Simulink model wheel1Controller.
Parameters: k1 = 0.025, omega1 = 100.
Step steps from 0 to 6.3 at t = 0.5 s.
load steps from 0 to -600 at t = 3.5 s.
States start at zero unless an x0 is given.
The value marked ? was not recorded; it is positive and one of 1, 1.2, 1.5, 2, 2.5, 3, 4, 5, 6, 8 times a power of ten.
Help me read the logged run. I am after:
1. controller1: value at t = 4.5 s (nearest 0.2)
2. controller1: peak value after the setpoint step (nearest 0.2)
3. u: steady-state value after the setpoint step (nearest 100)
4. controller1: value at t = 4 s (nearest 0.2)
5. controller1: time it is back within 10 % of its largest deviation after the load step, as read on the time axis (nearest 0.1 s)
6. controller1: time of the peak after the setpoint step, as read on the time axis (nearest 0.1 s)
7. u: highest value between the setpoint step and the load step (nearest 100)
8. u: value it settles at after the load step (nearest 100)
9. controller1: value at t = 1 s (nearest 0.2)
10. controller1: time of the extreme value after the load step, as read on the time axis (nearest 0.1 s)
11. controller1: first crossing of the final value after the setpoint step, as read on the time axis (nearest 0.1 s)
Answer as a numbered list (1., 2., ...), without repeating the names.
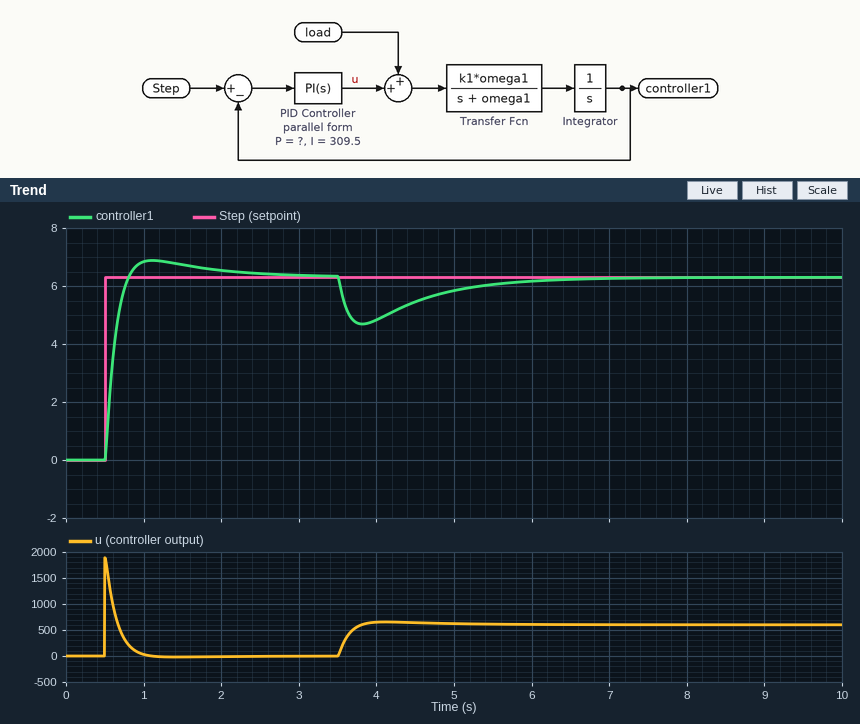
1. 5.4
2. 6.8
3. 0
4. 4.8
5. 5.8 s
6. 1.1 s
7. 1900
8. 600
9. 6.8
10. 3.8 s
11. 0.8 s
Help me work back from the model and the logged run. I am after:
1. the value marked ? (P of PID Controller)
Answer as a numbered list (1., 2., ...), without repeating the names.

1. 300
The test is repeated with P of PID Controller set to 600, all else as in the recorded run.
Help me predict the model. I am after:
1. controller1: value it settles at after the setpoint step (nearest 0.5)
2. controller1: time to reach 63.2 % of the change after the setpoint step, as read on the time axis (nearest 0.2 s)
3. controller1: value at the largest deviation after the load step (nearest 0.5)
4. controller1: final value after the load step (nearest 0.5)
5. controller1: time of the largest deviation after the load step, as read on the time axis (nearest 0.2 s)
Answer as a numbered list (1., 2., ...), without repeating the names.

1. 6.5
2. 0.6 s
3. 5.5
4. 6.5
5. 3.8 s
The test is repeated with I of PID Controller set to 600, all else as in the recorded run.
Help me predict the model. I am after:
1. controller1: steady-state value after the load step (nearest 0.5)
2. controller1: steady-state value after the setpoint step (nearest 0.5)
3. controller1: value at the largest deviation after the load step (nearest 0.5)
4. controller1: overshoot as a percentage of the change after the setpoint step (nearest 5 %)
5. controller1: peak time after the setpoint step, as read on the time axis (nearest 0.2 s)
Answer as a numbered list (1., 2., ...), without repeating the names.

1. 6.5
2. 6.5
3. 5.0
4. 15 %
5. 1.0 s
